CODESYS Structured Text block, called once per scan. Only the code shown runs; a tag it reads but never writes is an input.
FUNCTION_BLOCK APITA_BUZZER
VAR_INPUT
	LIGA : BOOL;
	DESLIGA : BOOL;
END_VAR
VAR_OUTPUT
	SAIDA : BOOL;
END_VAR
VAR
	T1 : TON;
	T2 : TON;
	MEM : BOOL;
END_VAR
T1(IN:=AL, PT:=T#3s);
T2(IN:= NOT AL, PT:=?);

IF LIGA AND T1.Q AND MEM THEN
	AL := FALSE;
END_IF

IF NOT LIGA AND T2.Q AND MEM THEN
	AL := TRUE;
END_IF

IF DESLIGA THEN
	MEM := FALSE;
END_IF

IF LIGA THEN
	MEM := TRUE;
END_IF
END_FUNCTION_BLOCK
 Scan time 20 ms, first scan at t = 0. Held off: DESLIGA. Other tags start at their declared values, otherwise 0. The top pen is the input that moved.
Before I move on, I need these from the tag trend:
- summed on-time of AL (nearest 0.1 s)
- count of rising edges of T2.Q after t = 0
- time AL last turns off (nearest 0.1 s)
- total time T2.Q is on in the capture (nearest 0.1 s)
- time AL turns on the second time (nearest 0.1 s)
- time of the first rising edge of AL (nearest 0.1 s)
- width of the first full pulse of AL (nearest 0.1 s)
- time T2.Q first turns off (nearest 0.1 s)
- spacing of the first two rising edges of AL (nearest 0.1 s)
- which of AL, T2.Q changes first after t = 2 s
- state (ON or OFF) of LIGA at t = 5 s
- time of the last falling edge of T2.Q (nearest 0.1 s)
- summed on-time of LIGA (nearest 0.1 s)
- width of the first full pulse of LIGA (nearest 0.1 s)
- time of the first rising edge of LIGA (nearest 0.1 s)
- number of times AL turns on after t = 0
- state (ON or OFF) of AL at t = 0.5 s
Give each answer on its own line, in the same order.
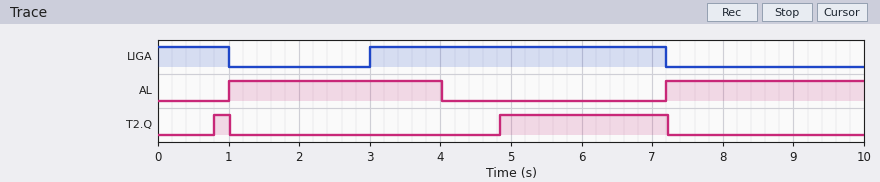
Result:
5.8 s
2
4.0 s
2.6 s
7.2 s
1.0 s
3.0 s
1.0 s
6.2 s
AL
ON
7.2 s
5.2 s
4.2 s
3.0 s
2
OFF
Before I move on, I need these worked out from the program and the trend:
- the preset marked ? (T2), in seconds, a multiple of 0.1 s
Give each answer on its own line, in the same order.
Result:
0.8 s
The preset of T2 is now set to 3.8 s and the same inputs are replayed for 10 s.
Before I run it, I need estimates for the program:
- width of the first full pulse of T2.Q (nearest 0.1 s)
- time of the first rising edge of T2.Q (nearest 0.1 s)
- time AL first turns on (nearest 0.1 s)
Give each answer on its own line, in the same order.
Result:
3.4 s
3.8 s
7.2 s
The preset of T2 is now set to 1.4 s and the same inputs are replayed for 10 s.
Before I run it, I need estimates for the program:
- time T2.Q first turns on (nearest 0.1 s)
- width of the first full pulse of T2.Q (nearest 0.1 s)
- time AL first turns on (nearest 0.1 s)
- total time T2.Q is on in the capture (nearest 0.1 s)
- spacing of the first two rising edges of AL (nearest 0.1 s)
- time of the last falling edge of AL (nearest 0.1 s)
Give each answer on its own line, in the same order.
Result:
1.4 s
0.0 s
1.4 s
1.4 s
5.8 s
4.4 s
